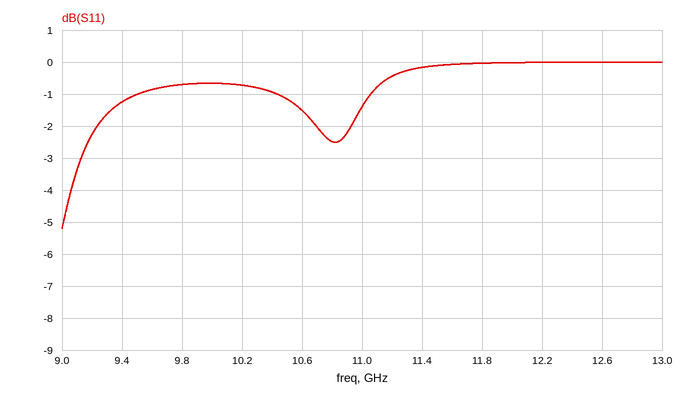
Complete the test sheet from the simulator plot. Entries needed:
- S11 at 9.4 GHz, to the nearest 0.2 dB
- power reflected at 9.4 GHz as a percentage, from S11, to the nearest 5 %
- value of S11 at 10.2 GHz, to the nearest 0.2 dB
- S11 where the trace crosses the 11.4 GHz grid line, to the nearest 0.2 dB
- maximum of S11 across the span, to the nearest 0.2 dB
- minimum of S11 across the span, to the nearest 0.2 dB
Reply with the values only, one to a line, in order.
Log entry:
-1.2 dB
75 %
-0.8 dB
-0.2 dB
0.0 dB
-5.2 dB
